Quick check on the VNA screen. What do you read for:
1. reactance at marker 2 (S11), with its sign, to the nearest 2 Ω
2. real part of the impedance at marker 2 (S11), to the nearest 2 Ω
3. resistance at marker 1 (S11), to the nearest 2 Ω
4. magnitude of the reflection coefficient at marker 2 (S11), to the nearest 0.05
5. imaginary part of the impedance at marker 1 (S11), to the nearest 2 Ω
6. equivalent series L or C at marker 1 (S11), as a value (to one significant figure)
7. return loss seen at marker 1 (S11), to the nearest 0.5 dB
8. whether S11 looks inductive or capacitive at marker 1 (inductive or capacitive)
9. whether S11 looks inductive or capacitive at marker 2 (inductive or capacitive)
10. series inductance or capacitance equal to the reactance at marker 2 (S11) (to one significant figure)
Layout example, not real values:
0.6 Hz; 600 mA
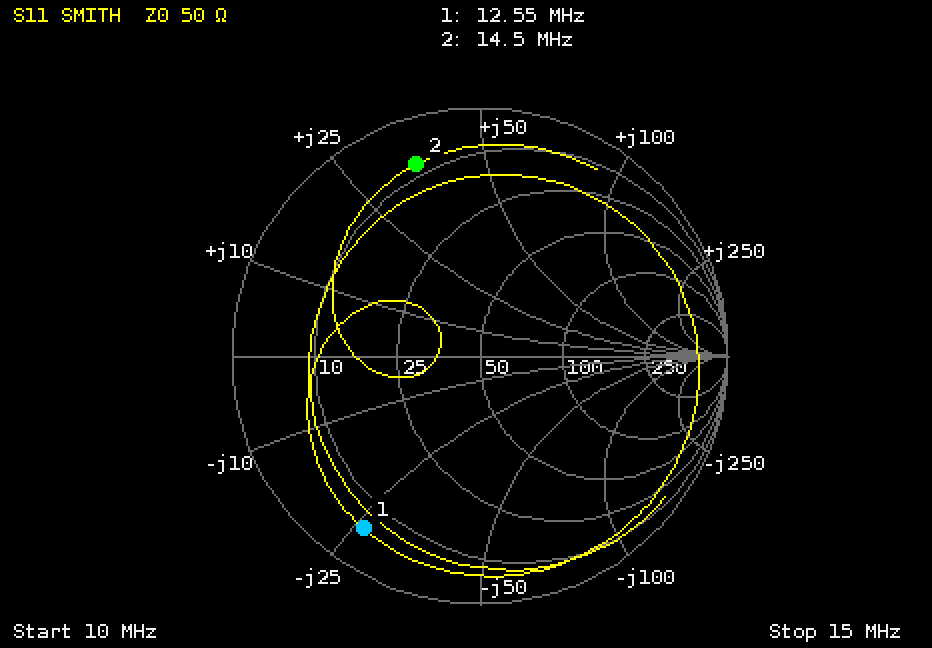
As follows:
+36 Ω; 8 Ω; 6 Ω; 0.80; -26 Ω; 500 pF; 1.5 dB; capacitive; inductive; 400 nH
